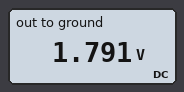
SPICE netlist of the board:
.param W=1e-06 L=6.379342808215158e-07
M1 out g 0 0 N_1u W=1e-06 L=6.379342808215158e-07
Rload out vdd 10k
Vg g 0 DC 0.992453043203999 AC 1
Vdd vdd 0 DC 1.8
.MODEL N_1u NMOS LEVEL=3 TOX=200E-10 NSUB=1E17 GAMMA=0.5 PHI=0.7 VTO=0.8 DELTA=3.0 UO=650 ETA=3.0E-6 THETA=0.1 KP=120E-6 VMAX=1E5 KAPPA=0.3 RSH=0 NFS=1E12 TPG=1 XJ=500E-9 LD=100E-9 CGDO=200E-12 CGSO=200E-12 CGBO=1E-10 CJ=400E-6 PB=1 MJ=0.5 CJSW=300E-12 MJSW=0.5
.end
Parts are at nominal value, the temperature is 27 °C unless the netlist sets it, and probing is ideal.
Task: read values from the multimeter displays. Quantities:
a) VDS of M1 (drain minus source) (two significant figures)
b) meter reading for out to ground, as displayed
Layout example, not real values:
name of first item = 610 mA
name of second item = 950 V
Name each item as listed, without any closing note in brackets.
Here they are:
VDS of M1 (drain minus source) = 1.8 V
meter reading for out to ground, as displayed = 1.791 V
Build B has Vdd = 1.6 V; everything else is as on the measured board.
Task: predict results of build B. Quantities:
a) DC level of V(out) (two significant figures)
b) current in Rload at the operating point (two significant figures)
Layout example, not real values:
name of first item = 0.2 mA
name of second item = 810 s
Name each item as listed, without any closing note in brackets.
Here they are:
DC level of V(out) = 1.6 V
current in Rload at the operating point = 900 nA
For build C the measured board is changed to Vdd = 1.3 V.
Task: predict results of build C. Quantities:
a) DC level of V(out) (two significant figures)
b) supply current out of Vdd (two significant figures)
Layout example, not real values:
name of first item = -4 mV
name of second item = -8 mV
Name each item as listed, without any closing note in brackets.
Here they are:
DC level of V(out) = 1.3 V
supply current out of Vdd = 880 nA
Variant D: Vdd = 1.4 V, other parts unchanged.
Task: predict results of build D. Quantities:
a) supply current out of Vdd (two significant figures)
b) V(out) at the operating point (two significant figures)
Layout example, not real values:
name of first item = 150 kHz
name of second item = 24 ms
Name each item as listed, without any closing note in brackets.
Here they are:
supply current out of Vdd = 890 nA
V(out) at the operating point = 1.4 V
